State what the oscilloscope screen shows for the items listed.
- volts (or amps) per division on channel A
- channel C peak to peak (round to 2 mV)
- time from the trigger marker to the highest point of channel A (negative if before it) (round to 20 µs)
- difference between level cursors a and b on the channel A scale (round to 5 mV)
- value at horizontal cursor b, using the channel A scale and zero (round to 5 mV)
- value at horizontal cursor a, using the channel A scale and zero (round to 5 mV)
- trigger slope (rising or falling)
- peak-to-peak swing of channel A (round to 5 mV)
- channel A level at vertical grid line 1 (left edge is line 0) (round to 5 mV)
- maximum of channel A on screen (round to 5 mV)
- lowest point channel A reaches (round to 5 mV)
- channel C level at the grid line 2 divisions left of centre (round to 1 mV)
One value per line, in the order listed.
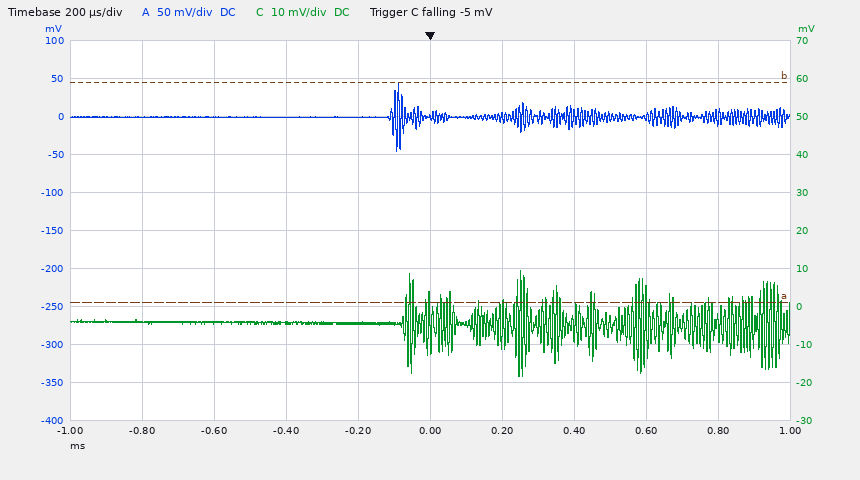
50 mV
28 mV
-80 µs
290 mV
45 mV
-245 mV
falling
90 mV
0 mV
45 mV
-45 mV
-4 mV
